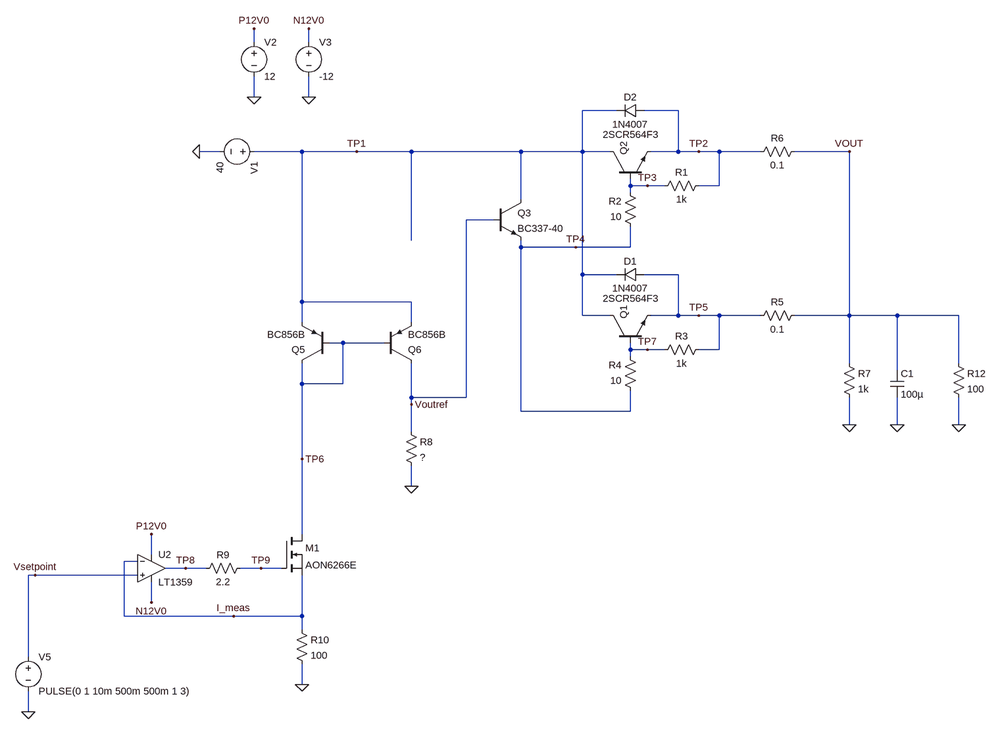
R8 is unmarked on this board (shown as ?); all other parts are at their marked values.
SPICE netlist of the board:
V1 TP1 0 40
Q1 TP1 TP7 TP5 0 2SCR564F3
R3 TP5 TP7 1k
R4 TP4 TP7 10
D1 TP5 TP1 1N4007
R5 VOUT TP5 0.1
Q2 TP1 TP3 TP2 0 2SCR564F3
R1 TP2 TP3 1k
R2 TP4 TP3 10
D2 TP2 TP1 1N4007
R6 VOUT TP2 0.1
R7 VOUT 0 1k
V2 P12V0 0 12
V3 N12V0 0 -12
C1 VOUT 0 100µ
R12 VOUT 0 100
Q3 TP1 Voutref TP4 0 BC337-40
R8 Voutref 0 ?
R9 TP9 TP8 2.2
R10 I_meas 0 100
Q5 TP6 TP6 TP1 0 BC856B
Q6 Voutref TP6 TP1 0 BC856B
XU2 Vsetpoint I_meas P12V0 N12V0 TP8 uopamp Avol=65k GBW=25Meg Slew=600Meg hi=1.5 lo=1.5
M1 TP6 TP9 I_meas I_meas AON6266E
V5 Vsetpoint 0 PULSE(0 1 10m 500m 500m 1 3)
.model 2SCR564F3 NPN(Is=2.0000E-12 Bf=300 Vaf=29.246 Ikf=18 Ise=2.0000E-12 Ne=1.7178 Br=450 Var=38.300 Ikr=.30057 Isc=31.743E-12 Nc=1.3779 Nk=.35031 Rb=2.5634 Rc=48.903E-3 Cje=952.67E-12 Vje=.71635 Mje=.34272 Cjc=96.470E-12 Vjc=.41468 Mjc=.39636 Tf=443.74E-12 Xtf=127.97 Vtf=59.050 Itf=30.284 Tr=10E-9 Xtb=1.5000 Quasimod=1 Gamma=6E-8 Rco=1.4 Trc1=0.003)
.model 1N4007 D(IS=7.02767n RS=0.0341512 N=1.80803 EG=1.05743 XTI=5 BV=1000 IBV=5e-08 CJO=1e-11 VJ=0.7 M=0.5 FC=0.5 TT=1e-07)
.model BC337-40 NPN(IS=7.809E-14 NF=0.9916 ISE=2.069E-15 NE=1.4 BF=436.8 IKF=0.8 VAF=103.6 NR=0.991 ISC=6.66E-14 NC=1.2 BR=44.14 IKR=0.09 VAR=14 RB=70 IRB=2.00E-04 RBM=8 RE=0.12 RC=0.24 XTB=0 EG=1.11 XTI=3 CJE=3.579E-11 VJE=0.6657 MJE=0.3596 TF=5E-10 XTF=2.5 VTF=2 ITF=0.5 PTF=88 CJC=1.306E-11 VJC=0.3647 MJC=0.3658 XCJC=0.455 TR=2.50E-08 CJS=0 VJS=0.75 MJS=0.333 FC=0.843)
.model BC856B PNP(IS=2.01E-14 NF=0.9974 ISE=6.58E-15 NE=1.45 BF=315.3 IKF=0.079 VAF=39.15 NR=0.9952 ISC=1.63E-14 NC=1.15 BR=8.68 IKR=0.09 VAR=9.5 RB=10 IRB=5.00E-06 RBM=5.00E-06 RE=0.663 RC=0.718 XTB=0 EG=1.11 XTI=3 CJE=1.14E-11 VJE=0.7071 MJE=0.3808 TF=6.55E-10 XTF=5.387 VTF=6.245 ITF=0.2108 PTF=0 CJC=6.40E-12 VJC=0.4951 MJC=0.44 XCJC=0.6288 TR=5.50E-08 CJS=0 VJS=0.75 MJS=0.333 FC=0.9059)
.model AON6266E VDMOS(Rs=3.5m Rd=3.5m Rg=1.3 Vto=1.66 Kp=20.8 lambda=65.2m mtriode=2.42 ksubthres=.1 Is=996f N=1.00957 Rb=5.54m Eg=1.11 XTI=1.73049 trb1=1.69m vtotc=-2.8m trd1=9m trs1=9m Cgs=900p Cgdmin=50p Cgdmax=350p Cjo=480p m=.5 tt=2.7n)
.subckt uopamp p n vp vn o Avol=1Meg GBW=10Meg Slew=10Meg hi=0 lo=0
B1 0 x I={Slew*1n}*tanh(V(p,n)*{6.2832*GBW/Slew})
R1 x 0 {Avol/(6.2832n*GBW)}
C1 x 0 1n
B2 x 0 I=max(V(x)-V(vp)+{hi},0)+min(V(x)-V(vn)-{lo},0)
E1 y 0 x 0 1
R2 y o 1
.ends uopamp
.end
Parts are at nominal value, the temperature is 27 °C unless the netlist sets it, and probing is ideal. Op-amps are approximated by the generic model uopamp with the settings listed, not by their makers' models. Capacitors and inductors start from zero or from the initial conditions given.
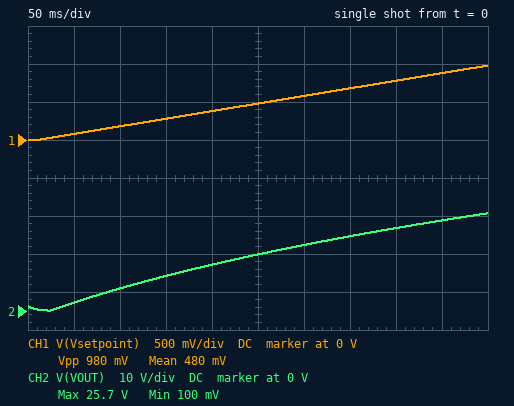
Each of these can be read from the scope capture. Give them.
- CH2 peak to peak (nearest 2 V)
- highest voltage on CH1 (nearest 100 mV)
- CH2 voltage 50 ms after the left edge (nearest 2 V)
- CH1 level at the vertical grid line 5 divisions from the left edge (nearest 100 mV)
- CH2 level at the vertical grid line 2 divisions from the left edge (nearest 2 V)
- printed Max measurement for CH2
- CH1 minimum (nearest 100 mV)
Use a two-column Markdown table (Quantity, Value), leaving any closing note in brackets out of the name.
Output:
| Quantity | Value |
|---|---|
| CH2 peak to peak | 26 V |
| highest voltage on CH1 | 1.0 V |
| CH2 voltage 50 ms after the left edge | 2 V |
| CH1 level at the vertical grid line 5 divisions from the left edge | 500 mV |
| CH2 level at the vertical grid line 2 divisions from the left edge | 6 V |
| printed Max measurement for CH2 | 25.7 V |
| CH1 minimum | 0 V |
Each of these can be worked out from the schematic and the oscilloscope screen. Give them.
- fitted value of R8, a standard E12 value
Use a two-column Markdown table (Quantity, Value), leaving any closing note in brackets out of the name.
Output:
| Quantity | Value |
|---|---|
| fitted value of R8, a standard E12 value | 2.2 kΩ |
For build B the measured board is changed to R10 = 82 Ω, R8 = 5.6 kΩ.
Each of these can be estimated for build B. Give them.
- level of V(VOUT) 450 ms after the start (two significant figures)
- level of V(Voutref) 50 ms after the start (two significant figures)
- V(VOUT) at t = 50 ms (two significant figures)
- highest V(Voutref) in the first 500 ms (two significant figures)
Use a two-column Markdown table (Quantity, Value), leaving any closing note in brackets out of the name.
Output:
| Quantity | Value |
|---|---|
| level of V(VOUT) 450 ms after the start | 39 V |
| level of V(Voutref) 50 ms after the start | 9.6 V |
| V(VOUT) at t = 50 ms | 8.4 V |
| highest V(Voutref) in the first 500 ms | 40 V |
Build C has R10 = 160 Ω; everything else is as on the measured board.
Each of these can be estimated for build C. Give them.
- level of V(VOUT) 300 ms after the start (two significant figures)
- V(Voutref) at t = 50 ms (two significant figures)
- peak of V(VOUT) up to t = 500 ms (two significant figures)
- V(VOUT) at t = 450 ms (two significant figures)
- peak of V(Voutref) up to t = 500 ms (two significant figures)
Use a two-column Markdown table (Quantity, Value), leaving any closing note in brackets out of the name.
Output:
| Quantity | Value |
|---|---|
| level of V(VOUT) 300 ms after the start | 12 V |
| V(Voutref) at t = 50 ms | 2.2 V |
| peak of V(VOUT) up to t = 500 ms | 18 V |
| V(VOUT) at t = 450 ms | 17 V |
| peak of V(Voutref) up to t = 500 ms | 19 V |
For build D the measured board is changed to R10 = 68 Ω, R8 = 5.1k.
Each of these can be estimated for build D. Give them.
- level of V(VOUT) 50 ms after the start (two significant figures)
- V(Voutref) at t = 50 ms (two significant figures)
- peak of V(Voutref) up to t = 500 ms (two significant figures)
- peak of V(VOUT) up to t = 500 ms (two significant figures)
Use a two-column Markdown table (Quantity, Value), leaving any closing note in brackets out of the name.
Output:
| Quantity | Value |
|---|---|
| level of V(VOUT) 50 ms after the start | 9.2 V |
| V(Voutref) at t = 50 ms | 10 V |
| peak of V(Voutref) up to t = 500 ms | 40 V |
| peak of V(VOUT) up to t = 500 ms | 39 V |
